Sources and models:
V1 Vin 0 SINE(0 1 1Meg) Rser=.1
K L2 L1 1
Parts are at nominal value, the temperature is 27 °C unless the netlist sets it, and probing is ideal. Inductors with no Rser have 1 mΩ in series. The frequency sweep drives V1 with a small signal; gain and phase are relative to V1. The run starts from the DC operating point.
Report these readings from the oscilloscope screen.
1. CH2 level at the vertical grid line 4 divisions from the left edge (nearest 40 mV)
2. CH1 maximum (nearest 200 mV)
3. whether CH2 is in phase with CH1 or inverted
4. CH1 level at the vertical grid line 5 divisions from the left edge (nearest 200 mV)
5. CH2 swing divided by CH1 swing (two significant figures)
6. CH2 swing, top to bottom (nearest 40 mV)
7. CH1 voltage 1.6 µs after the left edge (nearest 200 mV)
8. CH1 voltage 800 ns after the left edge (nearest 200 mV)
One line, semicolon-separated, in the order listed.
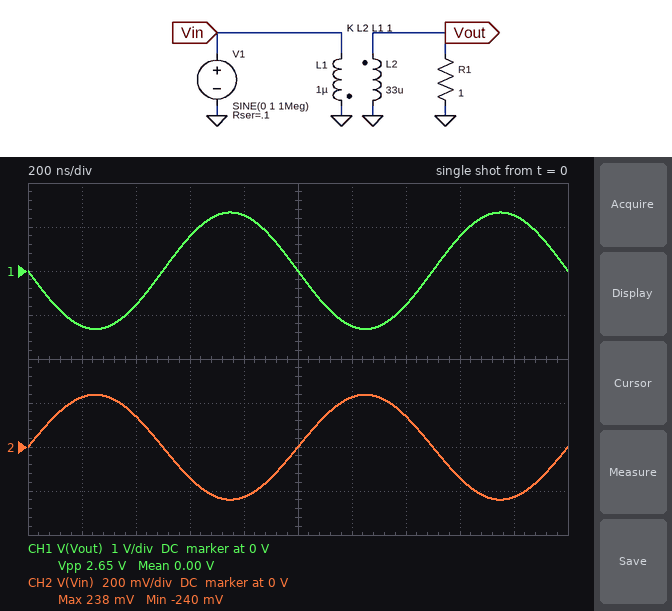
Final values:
-240 mV; 1.4 V; inverted; 0 V; 0.18; 480 mV; 800 mV; 1.2 V
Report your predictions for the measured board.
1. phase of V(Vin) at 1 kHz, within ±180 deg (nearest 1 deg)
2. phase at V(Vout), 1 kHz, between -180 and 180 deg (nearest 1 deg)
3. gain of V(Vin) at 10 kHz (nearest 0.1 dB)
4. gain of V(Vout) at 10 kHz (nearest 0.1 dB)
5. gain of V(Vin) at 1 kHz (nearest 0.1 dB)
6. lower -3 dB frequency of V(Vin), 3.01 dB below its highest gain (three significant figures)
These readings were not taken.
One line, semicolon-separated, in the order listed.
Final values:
66 deg; -105 deg; -13.0 dB; 1.9 dB; -24.0 dB; 3.71 kHz
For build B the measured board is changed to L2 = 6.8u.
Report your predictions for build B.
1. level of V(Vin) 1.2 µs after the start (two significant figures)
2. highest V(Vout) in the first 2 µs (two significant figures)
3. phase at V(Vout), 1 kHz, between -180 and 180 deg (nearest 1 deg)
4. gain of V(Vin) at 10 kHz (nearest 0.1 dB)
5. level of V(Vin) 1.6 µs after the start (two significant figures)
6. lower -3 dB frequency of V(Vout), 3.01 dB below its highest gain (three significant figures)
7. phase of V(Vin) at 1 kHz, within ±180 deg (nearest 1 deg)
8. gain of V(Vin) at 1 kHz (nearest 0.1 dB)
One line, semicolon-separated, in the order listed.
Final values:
560 mV; 1.6 V; -96 deg; -7.3 dB; -360 mV; 9.53 kHz; 75 deg; -24.0 dB
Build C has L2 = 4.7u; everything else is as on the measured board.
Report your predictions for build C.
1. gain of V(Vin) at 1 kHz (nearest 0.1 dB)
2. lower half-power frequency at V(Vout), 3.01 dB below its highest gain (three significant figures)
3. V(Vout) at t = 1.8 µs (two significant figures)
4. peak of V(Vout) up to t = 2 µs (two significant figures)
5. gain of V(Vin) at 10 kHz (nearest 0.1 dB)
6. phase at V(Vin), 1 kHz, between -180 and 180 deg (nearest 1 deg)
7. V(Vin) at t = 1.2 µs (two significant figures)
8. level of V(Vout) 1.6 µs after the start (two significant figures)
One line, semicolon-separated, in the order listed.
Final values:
-24.0 dB; 10.9 kHz; 1.4 V; 1.5 V; -6.7 dB; 76 deg; 640 mV; 890 mV
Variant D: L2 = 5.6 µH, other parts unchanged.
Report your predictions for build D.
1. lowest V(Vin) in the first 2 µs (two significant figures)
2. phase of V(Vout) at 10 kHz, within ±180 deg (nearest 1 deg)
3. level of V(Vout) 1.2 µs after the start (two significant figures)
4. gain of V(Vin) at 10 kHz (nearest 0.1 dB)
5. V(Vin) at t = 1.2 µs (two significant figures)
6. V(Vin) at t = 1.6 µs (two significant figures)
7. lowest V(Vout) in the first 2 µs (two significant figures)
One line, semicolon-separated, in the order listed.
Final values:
-650 mV; -134 deg; -1.4 V; -7.0 dB; 610 mV; -390 mV; -1.5 V
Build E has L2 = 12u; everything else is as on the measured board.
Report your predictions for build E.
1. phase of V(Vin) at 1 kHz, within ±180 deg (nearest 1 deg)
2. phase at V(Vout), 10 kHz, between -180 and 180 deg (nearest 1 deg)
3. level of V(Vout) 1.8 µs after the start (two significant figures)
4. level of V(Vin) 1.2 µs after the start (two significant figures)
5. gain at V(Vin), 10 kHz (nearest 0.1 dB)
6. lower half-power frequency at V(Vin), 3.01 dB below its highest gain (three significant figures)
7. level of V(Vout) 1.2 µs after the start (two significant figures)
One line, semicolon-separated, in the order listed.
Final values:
73 deg; -144 deg; 1.5 V; 430 mV; -8.6 dB; 7.27 kHz; -1.5 V
